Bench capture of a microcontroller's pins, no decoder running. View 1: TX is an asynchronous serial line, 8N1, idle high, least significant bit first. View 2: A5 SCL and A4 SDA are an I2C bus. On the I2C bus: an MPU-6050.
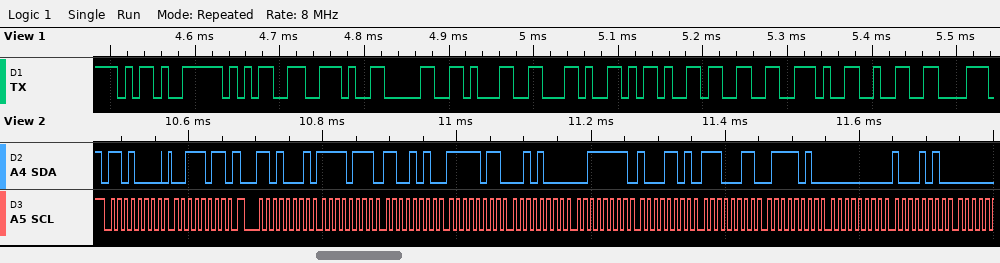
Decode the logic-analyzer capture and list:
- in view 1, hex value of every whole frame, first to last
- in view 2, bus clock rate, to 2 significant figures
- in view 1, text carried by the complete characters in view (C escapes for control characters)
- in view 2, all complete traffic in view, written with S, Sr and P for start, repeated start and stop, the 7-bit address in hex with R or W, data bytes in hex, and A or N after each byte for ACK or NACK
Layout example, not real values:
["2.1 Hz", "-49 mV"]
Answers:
["0x2D 0x35 0x2E 0x30 0x31 0x2C 0x2D 0x33 0x2E 0x32", "100 kHz", "\"-5.01,-3.2\"", "S 68W A 3B A Sr 68R A F7 A CA A FB A 28 A 3F A 8D A E3 A 7A A 00 A 8A A"]
